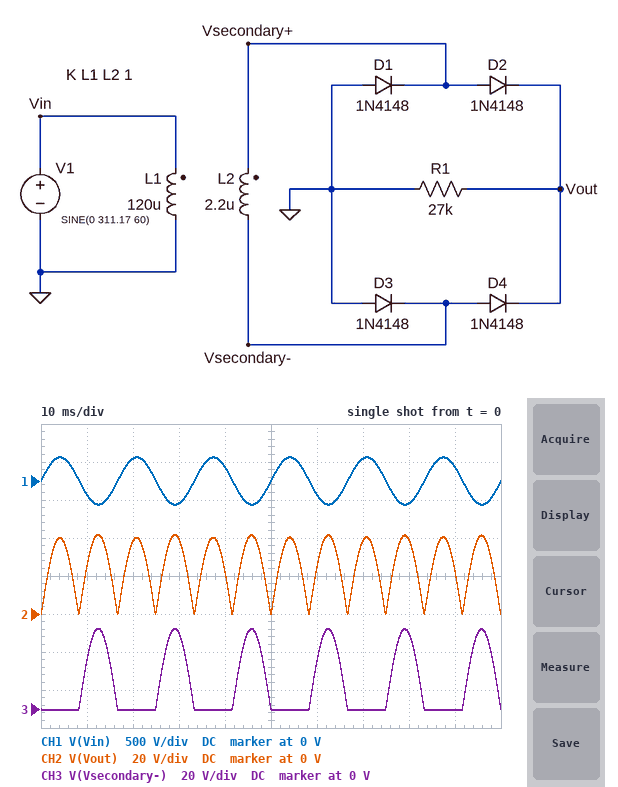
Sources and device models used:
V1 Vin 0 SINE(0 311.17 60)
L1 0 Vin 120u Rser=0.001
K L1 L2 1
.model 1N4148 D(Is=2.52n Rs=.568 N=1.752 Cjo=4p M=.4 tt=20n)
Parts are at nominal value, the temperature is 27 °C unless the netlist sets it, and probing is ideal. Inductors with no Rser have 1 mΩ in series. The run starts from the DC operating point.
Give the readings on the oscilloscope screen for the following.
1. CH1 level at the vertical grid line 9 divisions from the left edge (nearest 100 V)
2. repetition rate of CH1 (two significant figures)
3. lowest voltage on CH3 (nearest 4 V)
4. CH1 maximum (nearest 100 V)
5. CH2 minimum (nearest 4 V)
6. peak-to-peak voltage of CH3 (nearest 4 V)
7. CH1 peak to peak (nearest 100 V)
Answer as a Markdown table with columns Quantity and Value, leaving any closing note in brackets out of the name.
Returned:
| Quantity | Value |
|---|---|
| CH1 level at the vertical grid line 9 divisions from the left edge | 200 V |
| repetition rate of CH1 | 60 Hz |
| lowest voltage on CH3 | 0 V |
| CH1 maximum | 300 V |
| CH2 minimum | 0 V |
| peak-to-peak voltage of CH3 | 44 V |
| CH1 peak to peak | 600 V |
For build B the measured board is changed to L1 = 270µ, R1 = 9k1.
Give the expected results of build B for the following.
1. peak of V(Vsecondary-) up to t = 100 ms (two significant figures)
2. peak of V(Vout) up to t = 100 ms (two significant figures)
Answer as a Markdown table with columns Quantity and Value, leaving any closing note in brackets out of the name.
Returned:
| Quantity | Value |
|---|---|
| peak of V(Vsecondary-) up to t = 100 ms | 28 V |
| peak of V(Vout) up to t = 100 ms | 27 V |
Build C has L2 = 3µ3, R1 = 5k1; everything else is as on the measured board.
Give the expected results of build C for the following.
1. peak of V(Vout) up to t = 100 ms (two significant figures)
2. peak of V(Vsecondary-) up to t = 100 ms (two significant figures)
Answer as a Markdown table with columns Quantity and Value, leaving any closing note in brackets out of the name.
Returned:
| Quantity | Value |
|---|---|
| peak of V(Vout) up to t = 100 ms | 51 V |
| peak of V(Vsecondary-) up to t = 100 ms | 52 V |
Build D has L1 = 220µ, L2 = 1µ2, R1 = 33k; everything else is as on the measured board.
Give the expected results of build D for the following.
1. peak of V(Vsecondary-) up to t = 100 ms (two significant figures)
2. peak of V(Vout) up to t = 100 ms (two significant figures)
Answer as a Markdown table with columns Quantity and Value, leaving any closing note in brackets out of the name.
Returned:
| Quantity | Value |
|---|---|
| peak of V(Vsecondary-) up to t = 100 ms | 23 V |
| peak of V(Vout) up to t = 100 ms | 22 V |
